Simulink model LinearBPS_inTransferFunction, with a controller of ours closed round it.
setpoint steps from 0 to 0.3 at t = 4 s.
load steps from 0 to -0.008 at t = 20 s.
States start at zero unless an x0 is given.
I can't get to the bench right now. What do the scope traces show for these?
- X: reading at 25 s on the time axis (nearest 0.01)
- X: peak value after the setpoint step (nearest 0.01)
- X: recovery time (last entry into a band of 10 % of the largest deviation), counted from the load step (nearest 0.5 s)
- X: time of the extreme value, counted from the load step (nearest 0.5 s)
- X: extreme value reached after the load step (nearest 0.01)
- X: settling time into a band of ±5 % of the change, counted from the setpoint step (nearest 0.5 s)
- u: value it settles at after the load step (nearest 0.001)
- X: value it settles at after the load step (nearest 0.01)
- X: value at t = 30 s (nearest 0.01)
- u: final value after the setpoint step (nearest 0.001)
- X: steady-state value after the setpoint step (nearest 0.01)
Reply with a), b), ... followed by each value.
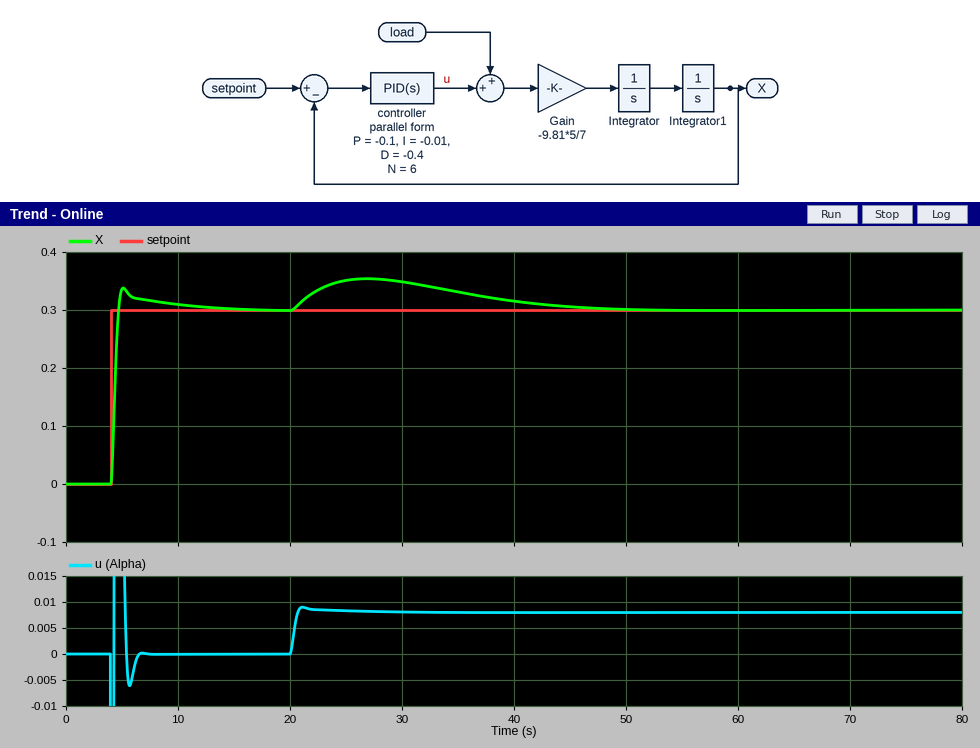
a) 0.35
b) 0.34
c) 25.0 s
d) 7.0 s
e) 0.35
f) 4.0 s
g) 0.008
h) 0.30
i) 0.35
j) 0.000
k) 0.30
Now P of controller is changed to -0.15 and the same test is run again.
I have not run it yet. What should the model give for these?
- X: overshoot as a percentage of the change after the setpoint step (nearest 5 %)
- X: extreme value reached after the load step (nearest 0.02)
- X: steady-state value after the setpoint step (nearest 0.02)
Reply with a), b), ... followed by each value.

a) 15 %
b) 0.34
c) 0.30
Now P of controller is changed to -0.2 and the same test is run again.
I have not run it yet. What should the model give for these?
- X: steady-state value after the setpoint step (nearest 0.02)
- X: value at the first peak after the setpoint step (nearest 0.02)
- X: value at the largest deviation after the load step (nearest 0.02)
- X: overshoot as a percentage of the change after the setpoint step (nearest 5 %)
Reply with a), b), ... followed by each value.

a) 0.30
b) 0.36
c) 0.34
d) 20 %
